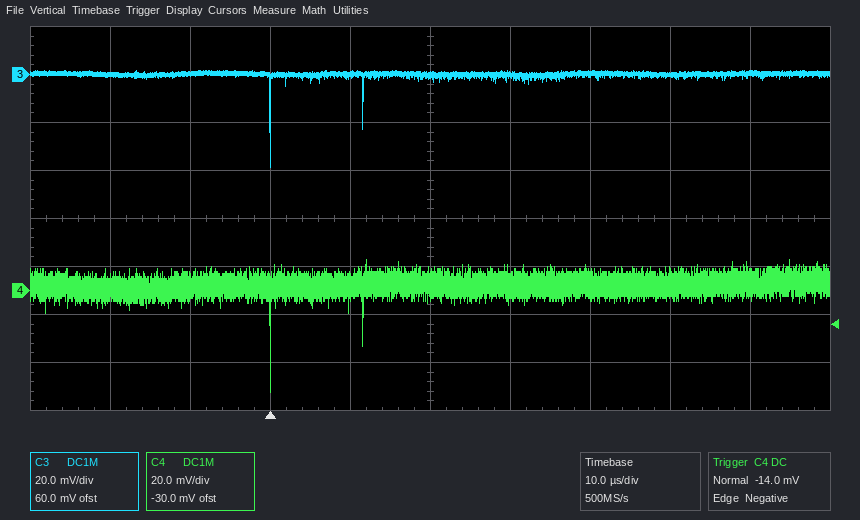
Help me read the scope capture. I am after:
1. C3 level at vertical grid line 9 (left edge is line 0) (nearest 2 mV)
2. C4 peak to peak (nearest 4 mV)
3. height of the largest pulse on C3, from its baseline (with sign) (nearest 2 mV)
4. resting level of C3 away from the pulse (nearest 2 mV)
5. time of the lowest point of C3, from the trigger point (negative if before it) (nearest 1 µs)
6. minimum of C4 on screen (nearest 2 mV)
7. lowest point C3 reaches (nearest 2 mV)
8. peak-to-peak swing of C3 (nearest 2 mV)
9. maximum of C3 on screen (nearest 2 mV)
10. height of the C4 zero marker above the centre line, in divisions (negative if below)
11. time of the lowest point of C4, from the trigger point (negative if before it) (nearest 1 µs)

0 mV
56 mV
-38 mV
0 mV
0 µs
-42 mV
-38 mV
40 mV
2 mV
-1.5 div
0 µs
